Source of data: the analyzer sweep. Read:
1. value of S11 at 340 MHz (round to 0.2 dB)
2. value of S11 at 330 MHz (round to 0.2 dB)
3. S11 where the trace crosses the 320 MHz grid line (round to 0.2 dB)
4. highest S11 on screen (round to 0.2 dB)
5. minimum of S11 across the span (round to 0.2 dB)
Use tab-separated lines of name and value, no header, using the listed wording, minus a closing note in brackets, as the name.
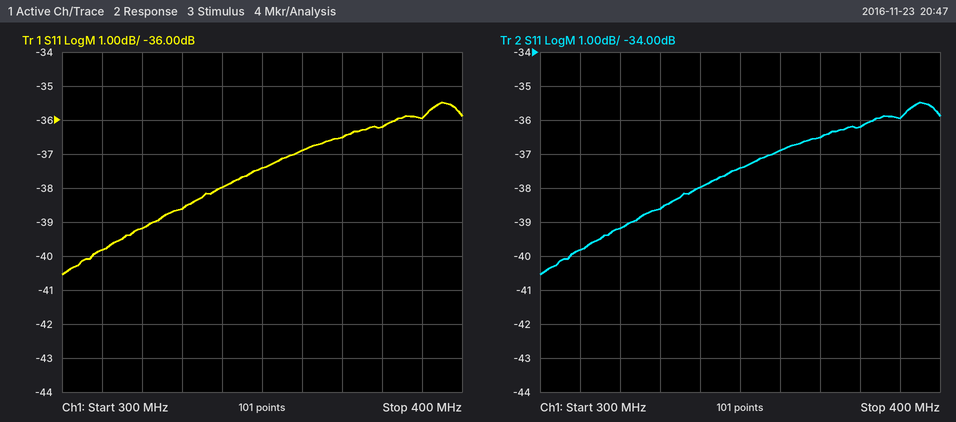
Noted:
value of S11 at 340 MHz	-38.0 dB
value of S11 at 330 MHz	-38.6 dB
S11 where the trace crosses the 320 MHz grid line	-39.2 dB
highest S11 on screen	-35.4 dB
minimum of S11 across the span	-40.6 dB
